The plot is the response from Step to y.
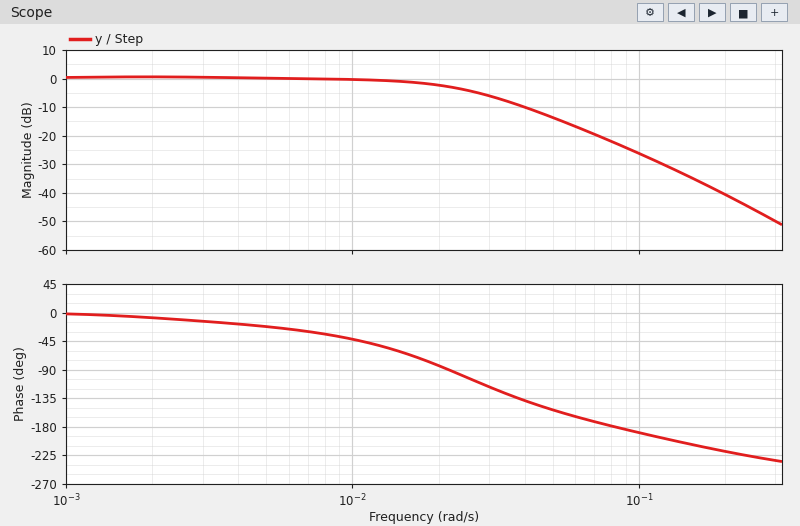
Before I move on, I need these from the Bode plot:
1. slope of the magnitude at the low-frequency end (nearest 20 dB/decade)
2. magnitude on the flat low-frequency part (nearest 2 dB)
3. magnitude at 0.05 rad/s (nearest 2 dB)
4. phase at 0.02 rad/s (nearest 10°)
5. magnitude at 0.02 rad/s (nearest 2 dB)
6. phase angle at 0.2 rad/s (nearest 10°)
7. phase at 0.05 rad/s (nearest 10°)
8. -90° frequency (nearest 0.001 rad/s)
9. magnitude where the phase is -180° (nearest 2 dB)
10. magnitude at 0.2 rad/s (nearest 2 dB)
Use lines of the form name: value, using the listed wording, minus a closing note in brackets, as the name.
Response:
slope of the magnitude at the low-frequency end: 0 dB/decade
magnitude on the flat low-frequency part: 0 dB
magnitude at 0.05 rad/s: -14 dB
phase at 0.02 rad/s: -80°
magnitude at 0.02 rad/s: -2 dB
phase angle at 0.2 rad/s: -220°
phase at 0.05 rad/s: -150°
-90° frequency: 0.022 rad/s
magnitude where the phase is -180°: -22 dB
magnitude at 0.2 rad/s: -40 dB
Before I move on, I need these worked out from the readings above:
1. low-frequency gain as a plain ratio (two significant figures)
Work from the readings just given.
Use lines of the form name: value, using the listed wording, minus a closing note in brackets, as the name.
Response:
low-frequency gain as a plain ratio: 1.0
